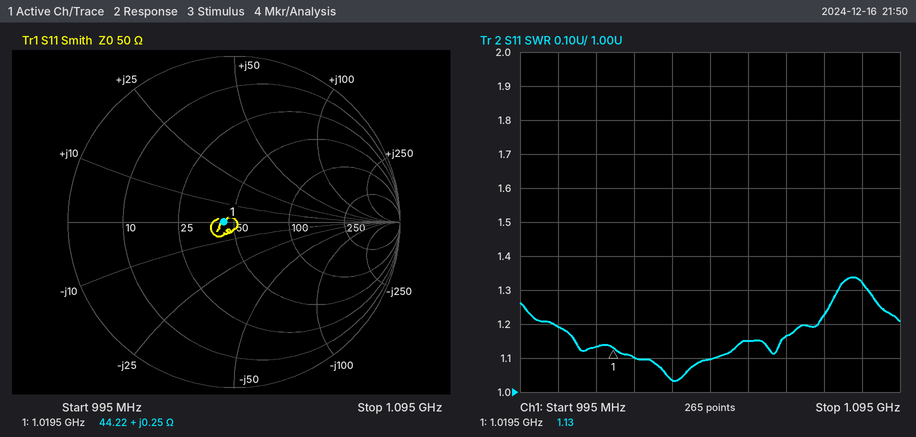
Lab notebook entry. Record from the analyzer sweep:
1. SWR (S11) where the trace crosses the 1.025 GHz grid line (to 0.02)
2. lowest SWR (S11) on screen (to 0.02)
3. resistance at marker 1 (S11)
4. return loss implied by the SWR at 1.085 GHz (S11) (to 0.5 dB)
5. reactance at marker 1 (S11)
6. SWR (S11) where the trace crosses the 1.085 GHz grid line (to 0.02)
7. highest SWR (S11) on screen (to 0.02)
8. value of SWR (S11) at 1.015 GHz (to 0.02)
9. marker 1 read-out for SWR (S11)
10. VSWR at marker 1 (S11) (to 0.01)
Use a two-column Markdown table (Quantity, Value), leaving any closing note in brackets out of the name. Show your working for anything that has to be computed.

| Quantity | Value |
|---|---|
| SWR (S11) where the trace crosses the 1.025 GHz grid line | 1.10 |
| lowest SWR (S11) on screen | 1.04 |
| resistance at marker 1 | 44.22 Ω |
| return loss implied by the SWR at 1.085 GHz (S11) | −20 log10((1.32 − 1)/(1.32 + 1)) ≈ 17.2 dB, so 17.0 dB to the nearest 0.5 dB |
| reactance at marker 1 | +0.25 Ω |
| SWR (S11) where the trace crosses the 1.085 GHz grid line | 1.32 |
| highest SWR (S11) on screen | 1.34 |
| value of SWR (S11) at 1.015 GHz | 1.14 |
| marker 1 read-out for SWR | 1.13 |
| VSWR at marker 1 (S11) | 1.13 |
